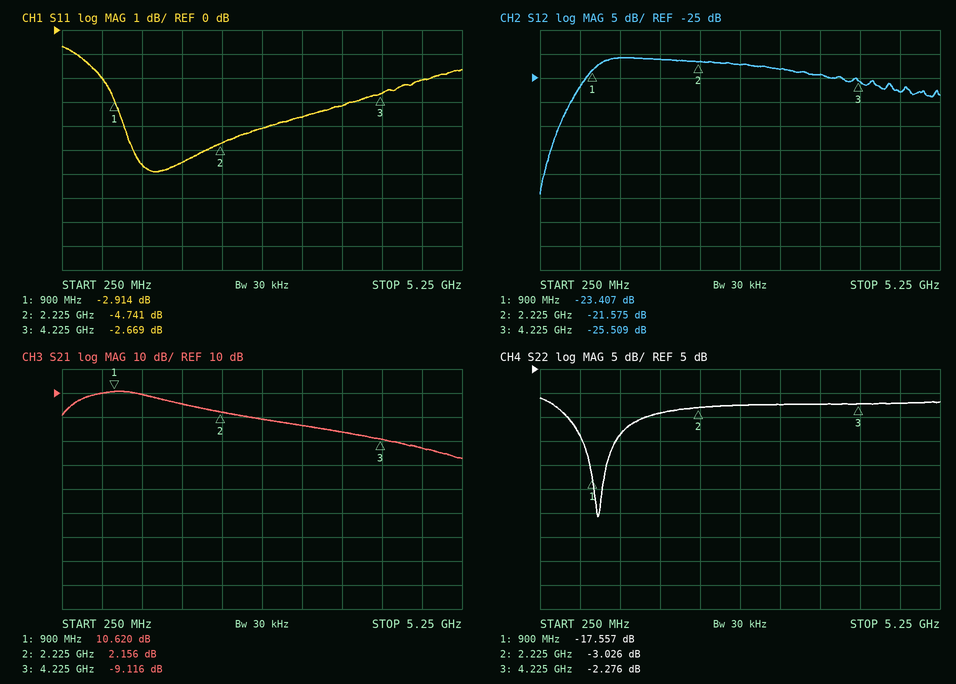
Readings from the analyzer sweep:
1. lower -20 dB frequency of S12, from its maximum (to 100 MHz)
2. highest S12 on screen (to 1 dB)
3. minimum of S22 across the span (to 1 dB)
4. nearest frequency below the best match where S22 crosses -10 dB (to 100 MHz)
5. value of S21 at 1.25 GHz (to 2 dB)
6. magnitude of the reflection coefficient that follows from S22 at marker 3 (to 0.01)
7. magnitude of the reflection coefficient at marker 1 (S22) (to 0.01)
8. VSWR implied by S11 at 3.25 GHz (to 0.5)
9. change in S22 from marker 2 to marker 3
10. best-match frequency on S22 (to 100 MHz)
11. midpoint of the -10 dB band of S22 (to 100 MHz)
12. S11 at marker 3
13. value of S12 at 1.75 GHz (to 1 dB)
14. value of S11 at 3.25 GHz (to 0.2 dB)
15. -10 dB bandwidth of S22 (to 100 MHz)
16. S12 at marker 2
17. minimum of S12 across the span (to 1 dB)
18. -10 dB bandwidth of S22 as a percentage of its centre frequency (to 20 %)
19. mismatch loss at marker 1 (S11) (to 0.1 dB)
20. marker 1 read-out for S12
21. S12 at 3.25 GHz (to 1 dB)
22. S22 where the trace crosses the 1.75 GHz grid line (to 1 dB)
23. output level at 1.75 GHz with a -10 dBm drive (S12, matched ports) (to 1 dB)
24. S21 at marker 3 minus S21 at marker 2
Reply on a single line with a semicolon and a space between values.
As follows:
400 MHz; -21 dB; -26 dB; 800 MHz; 10 dB; 0.77; 0.13; 5.0; 0.750 dB; 1.0 GHz; 1.0 GHz; -2.669 dB; -21 dB; -3.6 dB; 400 MHz; -21.575 dB; -49 dB; 40 %; 3.1 dB; -23.407 dB; -23 dB; -4 dB; -31 dBm; -11.272 dB
